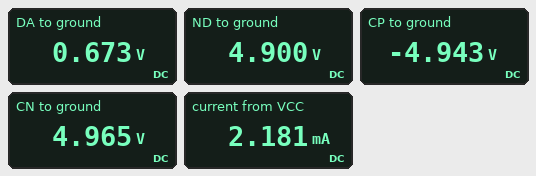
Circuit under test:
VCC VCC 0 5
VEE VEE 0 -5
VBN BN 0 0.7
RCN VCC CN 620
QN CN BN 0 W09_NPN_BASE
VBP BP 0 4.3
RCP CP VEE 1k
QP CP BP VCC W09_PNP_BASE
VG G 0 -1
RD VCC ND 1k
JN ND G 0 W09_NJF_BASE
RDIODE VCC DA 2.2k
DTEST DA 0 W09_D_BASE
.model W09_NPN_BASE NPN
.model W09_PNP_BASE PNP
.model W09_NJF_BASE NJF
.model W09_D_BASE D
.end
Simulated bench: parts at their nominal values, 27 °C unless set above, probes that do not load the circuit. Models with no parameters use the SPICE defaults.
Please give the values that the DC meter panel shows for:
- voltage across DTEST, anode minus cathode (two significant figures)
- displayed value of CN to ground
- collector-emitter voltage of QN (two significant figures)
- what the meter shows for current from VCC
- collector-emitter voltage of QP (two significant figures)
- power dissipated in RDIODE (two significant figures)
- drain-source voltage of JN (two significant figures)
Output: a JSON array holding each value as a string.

["670 mV", "4.965 V", "5.0 V", "2.181 mA", "-9.9 V", "8.5 mW", "4.9 V"]
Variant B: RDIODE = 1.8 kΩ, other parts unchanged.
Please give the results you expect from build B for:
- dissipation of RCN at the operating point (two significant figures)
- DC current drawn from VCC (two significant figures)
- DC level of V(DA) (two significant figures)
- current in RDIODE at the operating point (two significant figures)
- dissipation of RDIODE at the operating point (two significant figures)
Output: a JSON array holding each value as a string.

["2.0 µW", "2.6 mA", "680 mV", "2.4 mA", "10 mW"]
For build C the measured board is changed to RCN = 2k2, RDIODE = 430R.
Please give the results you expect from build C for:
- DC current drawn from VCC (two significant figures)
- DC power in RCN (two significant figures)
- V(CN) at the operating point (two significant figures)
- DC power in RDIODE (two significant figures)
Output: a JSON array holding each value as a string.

["10 mA", "7.1 µW", "4.9 V", "43 mW"]
